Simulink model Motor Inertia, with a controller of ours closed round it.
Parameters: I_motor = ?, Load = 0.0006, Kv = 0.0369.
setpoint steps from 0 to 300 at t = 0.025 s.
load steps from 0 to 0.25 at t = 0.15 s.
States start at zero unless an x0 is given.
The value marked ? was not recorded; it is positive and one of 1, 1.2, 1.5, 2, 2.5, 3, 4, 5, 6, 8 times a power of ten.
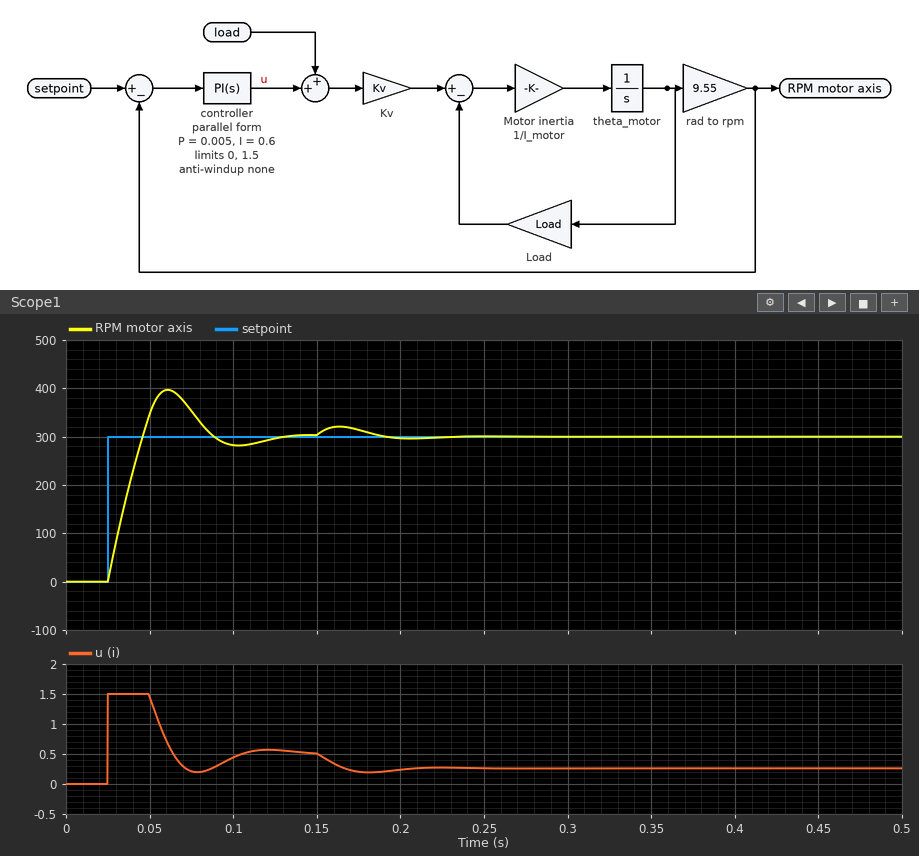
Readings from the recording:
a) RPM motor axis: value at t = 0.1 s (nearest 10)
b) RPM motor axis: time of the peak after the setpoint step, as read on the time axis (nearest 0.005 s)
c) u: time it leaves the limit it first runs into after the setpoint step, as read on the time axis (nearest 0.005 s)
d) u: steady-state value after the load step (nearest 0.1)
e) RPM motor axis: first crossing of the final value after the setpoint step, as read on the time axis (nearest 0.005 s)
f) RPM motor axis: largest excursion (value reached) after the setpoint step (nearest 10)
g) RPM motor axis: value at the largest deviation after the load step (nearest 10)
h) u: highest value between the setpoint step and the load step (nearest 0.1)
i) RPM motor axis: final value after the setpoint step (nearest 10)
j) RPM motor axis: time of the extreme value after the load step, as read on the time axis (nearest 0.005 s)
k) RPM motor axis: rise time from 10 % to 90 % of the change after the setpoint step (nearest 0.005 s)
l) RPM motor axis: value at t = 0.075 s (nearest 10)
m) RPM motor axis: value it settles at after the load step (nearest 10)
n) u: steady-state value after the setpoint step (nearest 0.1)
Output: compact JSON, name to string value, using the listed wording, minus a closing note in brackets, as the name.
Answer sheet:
{"RPM motor axis: value at t = 0.1 s": "280", "RPM motor axis: time of the peak after the setpoint step, as read on the time axis": "0.060 s", "u: time it leaves the limit it first runs into after the setpoint step, as read on the time axis": "0.050 s", "u: steady-state value after the load step": "0.3", "RPM motor axis: first crossing of the final value after the setpoint step, as read on the time axis": "0.045 s", "RPM motor axis: largest excursion (value reached) after the setpoint step": "400", "RPM motor axis: value at the largest deviation after the load step": "320", "u: highest value between the setpoint step and the load step": "1.5", "RPM motor axis: final value after the setpoint step": "300", "RPM motor axis: time of the extreme value after the load step, as read on the time axis": "0.165 s", "RPM motor axis: rise time from 10 % to 90 % of the change after the setpoint step": "0.015 s", "RPM motor axis: value at t = 0.075 s": "350", "RPM motor axis: value it settles at after the load step": "300", "u: steady-state value after the setpoint step": "0.5"}
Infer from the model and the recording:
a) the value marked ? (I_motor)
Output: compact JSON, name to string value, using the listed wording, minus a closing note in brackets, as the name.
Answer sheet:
{"the value marked ?": "3e-05"}
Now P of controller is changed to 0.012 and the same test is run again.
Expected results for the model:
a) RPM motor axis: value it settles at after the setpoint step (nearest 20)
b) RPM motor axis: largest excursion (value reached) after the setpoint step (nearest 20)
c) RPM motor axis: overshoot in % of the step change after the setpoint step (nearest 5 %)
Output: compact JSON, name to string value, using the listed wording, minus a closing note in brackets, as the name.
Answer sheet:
{"RPM motor axis: value it settles at after the setpoint step": "300", "RPM motor axis: largest excursion (value reached) after the setpoint step": "360", "RPM motor axis: overshoot in % of the step change after the setpoint step": "20 %"}
